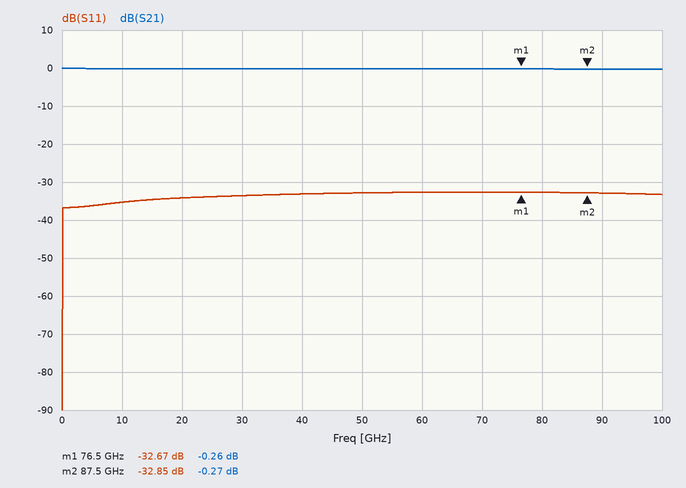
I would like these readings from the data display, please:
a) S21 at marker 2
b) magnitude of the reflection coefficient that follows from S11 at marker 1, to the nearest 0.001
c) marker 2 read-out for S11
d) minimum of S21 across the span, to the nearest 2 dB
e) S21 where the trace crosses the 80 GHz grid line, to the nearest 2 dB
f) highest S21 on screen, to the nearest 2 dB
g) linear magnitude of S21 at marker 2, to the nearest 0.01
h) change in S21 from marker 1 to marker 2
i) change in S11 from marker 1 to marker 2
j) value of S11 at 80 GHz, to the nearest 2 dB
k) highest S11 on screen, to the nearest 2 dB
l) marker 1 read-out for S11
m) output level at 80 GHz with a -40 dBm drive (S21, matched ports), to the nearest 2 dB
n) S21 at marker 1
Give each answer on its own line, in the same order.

-0.27 dB
0.023
-32.85 dB
0 dB
0 dB
0 dB
0.97
-0.01 dB
-0.18 dB
-32 dB
-32 dB
-32.67 dB
-40 dBm
-0.26 dB
